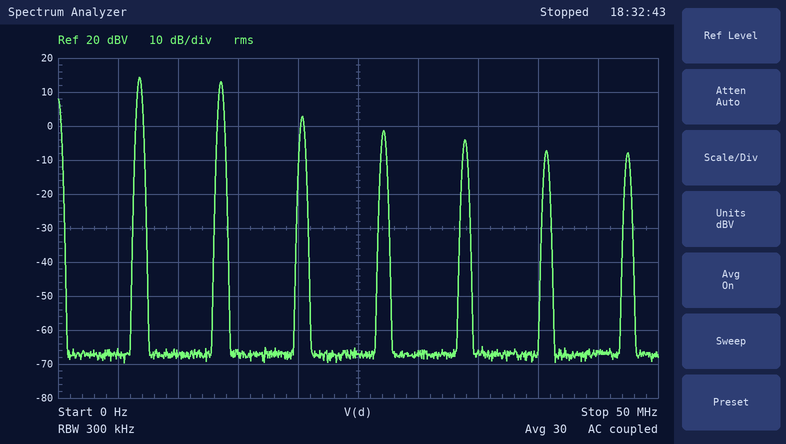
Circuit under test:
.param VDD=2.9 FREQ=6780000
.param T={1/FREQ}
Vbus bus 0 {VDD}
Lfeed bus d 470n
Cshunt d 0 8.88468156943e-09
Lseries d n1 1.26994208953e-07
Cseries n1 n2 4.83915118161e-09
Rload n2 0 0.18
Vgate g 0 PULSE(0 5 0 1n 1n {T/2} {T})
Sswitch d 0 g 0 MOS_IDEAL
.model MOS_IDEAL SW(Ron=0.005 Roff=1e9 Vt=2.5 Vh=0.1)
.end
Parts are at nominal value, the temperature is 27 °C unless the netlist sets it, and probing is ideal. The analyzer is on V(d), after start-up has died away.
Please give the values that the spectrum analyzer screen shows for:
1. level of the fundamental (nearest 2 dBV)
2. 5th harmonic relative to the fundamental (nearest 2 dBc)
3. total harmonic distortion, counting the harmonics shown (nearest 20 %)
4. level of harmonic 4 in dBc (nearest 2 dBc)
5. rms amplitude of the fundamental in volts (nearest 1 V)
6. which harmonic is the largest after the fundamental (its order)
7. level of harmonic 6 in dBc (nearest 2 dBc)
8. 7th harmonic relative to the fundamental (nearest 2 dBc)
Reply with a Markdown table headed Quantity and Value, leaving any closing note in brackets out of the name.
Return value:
| Quantity | Value |
|---|---|
| level of the fundamental | 14 dBV |
| 5th harmonic relative to the fundamental | -18 dBc |
| total harmonic distortion, counting the harmonics shown | 100 % |
| level of harmonic 4 in dBc | -16 dBc |
| rms amplitude of the fundamental in volts | 5 V |
| which harmonic is the largest after the fundamental | 2 |
| level of harmonic 6 in dBc | -22 dBc |
| 7th harmonic relative to the fundamental | -22 dBc |
